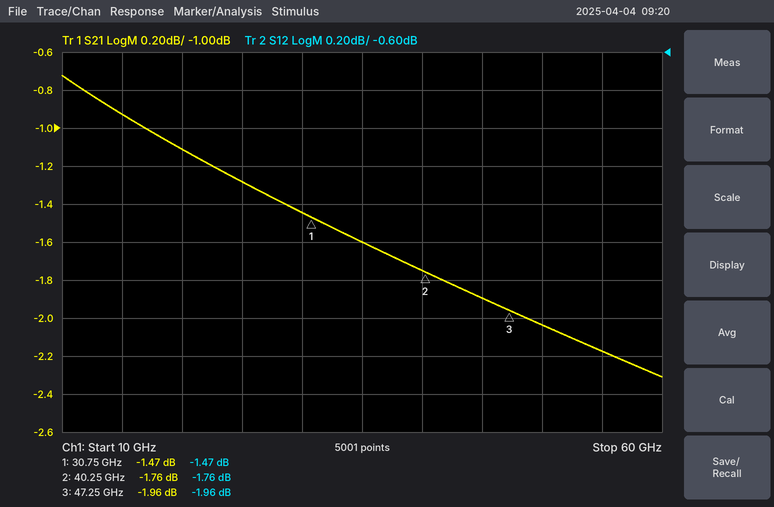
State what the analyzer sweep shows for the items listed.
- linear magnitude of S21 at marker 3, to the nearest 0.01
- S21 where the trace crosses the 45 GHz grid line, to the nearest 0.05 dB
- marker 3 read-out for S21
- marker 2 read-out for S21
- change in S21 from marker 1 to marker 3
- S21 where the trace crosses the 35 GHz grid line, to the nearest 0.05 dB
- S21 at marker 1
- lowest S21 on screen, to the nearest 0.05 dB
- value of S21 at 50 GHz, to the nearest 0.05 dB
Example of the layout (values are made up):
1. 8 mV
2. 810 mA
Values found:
1. 0.80
2. -1.90 dB
3. -1.96 dB
4. -1.76 dB
5. -0.49 dB
6. -1.60 dB
7. -1.47 dB
8. -2.30 dB
9. -2.05 dB
